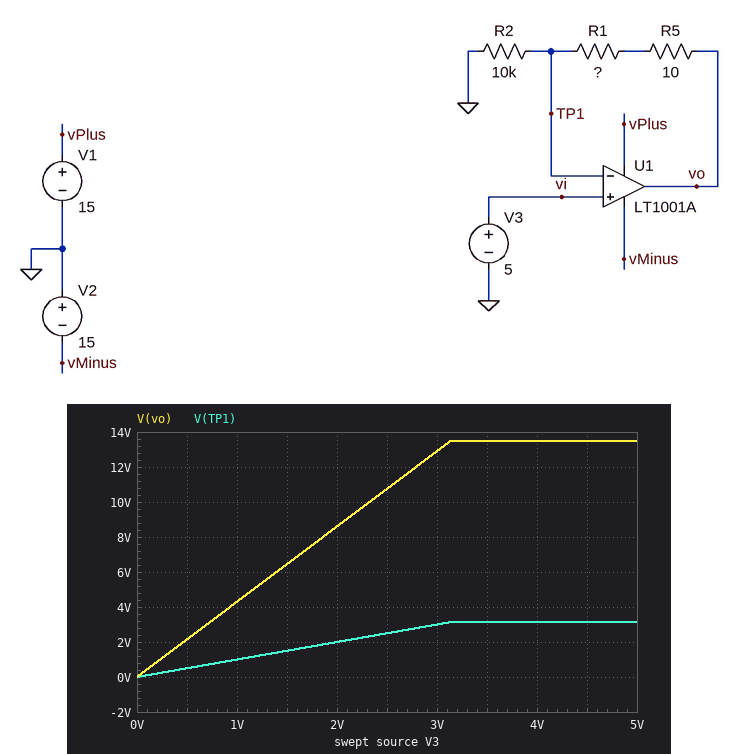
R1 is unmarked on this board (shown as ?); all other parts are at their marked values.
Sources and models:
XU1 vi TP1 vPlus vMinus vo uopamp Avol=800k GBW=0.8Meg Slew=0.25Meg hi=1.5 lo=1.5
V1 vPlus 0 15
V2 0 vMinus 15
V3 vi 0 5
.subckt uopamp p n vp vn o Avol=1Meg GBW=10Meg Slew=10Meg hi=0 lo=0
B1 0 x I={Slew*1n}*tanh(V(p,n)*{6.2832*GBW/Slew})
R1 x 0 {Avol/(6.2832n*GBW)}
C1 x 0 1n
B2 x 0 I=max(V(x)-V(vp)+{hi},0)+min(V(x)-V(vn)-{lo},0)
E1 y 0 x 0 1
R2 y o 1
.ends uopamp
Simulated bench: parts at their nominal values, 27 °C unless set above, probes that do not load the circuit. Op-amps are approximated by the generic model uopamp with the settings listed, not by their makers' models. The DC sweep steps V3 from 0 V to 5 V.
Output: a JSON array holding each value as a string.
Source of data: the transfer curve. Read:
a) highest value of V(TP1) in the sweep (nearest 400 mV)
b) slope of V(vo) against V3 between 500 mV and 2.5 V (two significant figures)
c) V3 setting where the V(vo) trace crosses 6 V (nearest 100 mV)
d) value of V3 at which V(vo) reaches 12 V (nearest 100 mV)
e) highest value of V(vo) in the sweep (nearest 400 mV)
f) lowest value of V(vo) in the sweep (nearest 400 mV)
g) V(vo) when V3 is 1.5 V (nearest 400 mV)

["3.2 V", "4.3 V/V", "1.4 V", "2.8 V", "13.6 V", "0 V", "6.4 V"]
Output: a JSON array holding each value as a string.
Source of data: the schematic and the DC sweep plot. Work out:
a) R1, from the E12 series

["33 kΩ"]
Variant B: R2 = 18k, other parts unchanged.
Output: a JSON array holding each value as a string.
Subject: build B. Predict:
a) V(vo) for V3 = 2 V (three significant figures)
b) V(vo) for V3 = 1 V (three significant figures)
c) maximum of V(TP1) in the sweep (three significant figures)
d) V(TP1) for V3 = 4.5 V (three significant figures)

["5.67 V", "2.83 V", "4.76 V", "4.50 V"]
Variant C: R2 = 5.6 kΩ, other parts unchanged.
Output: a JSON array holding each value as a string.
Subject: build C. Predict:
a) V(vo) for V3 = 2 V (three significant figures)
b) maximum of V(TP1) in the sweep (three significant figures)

["13.5 V", "1.96 V"]
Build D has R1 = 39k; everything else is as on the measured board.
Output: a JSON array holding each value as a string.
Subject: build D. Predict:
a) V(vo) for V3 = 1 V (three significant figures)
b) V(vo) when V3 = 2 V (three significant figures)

["4.90 V", "9.80 V"]
